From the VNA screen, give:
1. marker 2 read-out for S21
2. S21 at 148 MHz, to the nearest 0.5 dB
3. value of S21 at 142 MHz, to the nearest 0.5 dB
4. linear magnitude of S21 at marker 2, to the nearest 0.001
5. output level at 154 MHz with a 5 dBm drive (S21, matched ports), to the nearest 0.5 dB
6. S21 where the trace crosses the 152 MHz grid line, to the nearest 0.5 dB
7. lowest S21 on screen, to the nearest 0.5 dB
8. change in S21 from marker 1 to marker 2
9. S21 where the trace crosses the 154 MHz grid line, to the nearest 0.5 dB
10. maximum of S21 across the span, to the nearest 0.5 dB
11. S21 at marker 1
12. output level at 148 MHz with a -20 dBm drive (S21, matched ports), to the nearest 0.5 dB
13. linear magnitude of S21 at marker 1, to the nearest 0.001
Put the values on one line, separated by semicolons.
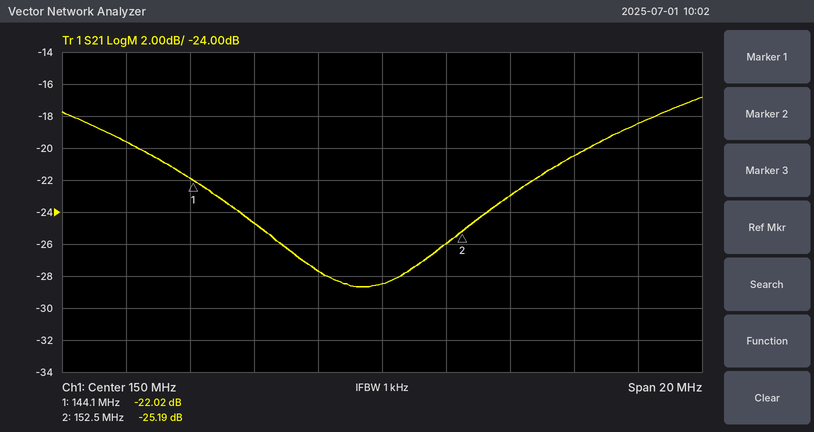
-25.19 dB; -27.5 dB; -19.5 dB; 0.055; -18.0 dBm; -26.0 dB; -28.5 dB; -3.17 dB; -23.0 dB; -17.0 dB; -22.02 dB; -47.5 dBm; 0.079
